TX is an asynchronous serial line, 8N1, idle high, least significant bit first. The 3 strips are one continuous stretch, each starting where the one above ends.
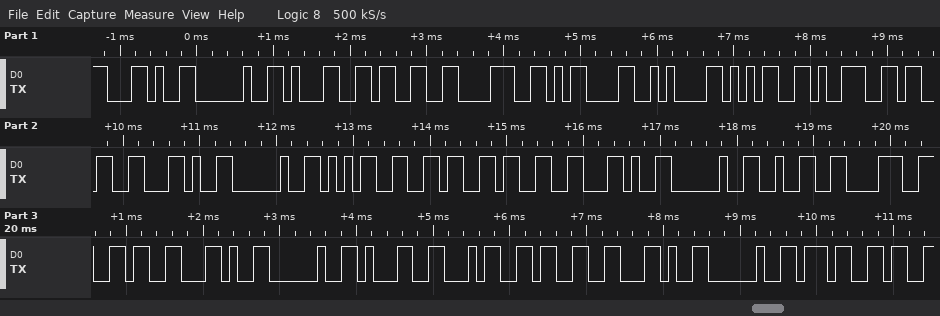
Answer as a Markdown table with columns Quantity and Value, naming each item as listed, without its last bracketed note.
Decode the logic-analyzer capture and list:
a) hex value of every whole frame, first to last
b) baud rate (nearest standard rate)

| Quantity | Value |
|---|---|
| hex value of every whole frame, first to last | 0x2C 0x20 0x31 0x33 0x38 0x0D 0x0A 0x35 0x39 0x33 0x2C 0x20 0x35 0x36 0x33 0x2C 0x20 0x32 0x38 0x36 0x2C 0x20 0x31 0x34 0x33 0x2C 0x20 0x37 |
| baud rate | 9600 baud |
